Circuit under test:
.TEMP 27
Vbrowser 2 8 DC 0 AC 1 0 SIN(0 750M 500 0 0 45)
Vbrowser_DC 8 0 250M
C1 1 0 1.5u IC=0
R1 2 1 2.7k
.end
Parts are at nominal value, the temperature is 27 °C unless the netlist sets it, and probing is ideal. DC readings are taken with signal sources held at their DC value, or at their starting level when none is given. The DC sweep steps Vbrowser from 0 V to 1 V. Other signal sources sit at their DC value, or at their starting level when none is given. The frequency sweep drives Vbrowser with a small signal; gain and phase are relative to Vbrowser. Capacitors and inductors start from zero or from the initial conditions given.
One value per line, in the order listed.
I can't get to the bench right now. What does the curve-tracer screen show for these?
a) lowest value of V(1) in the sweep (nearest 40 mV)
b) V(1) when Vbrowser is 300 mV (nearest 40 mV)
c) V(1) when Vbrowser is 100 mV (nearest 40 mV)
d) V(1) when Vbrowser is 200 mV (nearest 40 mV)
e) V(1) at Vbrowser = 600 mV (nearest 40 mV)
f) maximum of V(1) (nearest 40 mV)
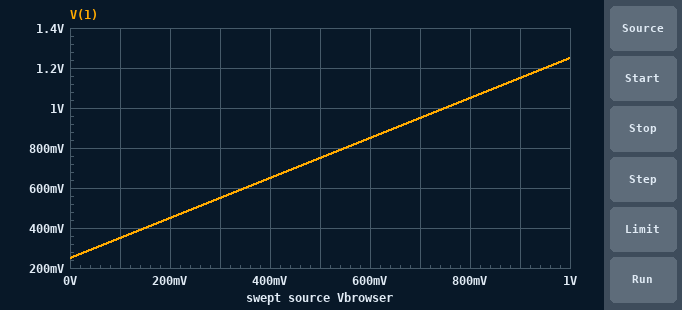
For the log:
240 mV
560 mV
360 mV
440 mV
840 mV
1.24 V
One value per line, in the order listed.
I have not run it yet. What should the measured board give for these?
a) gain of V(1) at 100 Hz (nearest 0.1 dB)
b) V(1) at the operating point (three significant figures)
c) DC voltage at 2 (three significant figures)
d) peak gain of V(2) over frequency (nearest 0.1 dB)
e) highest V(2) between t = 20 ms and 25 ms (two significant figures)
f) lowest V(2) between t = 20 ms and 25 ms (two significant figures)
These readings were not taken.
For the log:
-8.7 dB
250 mV
250 mV
0 dB
1.0 V
-500 mV
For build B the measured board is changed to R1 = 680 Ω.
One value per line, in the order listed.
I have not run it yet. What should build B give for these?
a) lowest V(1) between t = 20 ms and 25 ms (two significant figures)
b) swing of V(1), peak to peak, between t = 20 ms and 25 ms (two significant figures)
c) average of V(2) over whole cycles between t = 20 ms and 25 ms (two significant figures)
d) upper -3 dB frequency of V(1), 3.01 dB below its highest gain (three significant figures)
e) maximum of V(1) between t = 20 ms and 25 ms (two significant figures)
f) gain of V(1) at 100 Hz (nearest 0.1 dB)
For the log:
27 mV
450 mV
250 mV
156 Hz
470 mV
-1.5 dB
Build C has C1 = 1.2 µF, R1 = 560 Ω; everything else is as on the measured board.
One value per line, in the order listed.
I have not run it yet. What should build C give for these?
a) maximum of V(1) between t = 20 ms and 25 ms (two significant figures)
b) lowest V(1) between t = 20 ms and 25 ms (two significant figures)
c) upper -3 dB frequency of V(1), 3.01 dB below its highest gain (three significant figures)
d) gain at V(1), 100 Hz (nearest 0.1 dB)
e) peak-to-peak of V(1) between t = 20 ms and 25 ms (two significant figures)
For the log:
570 mV
-71 mV
237 Hz
-0.7 dB
640 mV
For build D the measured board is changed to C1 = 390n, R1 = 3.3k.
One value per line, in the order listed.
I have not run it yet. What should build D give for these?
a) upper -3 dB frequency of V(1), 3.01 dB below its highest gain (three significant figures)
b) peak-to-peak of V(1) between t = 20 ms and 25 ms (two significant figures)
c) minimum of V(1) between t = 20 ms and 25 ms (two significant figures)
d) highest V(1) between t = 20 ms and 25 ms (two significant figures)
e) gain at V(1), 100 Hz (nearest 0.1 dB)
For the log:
124 Hz
360 mV
70 mV
430 mV
-2.2 dB
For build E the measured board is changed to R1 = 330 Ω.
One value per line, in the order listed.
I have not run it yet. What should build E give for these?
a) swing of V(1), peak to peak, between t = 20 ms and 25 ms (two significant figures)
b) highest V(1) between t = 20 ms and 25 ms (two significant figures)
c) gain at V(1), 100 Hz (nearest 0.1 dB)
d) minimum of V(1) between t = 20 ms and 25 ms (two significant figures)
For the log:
810 mV
660 mV
-0.4 dB
-160 mV
